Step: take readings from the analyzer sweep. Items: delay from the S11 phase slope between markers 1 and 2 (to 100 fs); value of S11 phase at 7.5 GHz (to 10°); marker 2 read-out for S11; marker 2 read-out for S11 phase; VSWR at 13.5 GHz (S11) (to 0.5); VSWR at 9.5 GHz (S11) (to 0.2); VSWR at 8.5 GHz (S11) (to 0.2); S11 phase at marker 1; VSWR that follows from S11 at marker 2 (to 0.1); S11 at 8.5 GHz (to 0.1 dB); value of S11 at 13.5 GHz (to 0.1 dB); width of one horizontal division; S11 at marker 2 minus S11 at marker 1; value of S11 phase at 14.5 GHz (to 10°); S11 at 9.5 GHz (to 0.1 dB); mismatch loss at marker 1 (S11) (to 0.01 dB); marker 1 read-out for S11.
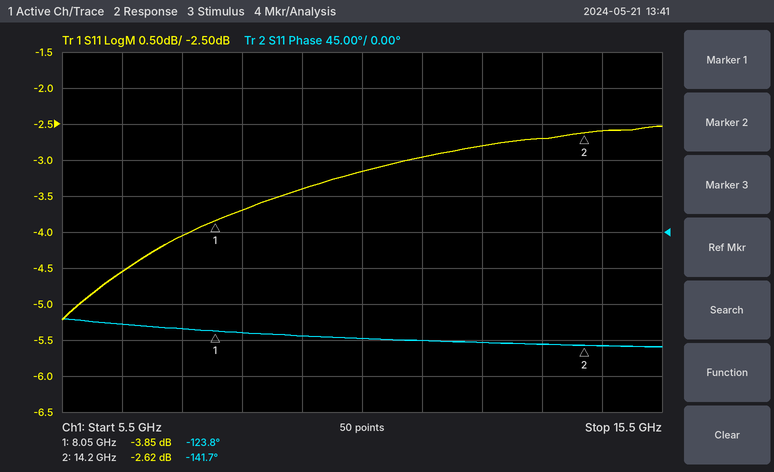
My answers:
8.1 ps
-120°
-2.62 dB
-141.7°
6.5
5.2
4.8
-123.8°
6.7
-3.7 dB
-2.7 dB
1 GHz
1.23 dB
-140°
-3.4 dB
2.31 dB
-3.85 dB
